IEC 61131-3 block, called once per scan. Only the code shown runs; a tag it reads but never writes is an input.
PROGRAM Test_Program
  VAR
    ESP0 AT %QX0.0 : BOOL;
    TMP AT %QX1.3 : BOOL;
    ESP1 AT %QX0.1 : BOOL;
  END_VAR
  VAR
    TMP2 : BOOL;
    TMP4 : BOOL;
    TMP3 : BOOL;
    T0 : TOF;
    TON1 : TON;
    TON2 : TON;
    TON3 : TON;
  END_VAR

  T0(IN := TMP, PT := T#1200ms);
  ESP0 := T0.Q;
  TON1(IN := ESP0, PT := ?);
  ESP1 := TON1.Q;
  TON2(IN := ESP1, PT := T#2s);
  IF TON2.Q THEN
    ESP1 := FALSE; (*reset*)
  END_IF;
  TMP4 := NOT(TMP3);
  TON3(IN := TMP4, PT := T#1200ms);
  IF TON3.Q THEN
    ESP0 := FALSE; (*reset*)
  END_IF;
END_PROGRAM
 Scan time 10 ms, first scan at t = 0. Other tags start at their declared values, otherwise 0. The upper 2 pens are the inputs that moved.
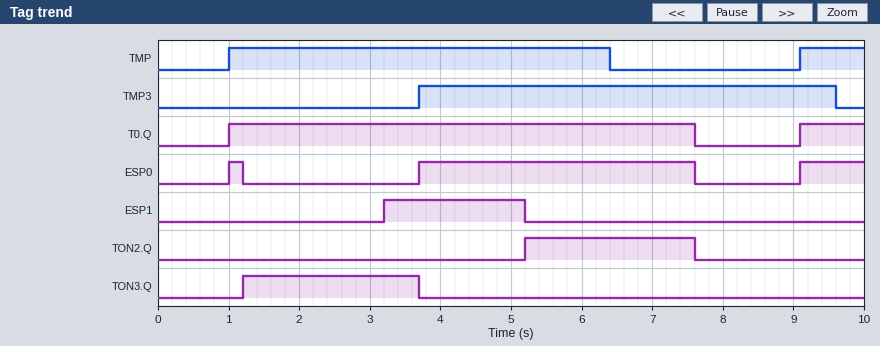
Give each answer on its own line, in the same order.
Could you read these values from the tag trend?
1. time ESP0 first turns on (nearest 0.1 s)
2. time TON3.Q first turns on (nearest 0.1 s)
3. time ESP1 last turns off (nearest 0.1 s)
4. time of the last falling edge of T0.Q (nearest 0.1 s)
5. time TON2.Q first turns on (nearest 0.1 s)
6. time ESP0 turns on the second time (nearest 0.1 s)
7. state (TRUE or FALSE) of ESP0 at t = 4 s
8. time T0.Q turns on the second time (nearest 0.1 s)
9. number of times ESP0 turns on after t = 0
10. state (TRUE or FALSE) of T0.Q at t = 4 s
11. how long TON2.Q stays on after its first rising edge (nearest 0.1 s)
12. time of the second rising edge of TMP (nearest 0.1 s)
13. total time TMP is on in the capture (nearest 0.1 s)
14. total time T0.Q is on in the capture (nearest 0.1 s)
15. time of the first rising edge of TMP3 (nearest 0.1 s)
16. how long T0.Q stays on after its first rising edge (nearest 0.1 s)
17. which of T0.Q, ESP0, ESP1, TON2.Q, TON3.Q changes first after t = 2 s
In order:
1.0 s
1.2 s
5.2 s
7.6 s
5.2 s
3.7 s
TRUE
9.1 s
3
TRUE
2.4 s
9.1 s
6.3 s
7.5 s
3.7 s
6.6 s
ESP1
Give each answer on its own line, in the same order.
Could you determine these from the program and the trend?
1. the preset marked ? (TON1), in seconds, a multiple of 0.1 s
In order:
2.2 s
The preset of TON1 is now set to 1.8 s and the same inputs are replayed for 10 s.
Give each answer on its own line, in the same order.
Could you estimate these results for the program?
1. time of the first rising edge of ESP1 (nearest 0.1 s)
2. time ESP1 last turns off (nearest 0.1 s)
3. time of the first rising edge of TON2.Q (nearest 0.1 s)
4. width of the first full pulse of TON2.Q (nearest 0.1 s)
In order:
2.8 s
4.8 s
4.8 s
2.8 s
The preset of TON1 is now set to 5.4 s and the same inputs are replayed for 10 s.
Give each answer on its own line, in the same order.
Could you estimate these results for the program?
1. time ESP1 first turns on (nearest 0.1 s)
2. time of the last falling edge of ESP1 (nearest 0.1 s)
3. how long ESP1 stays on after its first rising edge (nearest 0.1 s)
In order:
6.4 s
7.6 s
1.2 s
